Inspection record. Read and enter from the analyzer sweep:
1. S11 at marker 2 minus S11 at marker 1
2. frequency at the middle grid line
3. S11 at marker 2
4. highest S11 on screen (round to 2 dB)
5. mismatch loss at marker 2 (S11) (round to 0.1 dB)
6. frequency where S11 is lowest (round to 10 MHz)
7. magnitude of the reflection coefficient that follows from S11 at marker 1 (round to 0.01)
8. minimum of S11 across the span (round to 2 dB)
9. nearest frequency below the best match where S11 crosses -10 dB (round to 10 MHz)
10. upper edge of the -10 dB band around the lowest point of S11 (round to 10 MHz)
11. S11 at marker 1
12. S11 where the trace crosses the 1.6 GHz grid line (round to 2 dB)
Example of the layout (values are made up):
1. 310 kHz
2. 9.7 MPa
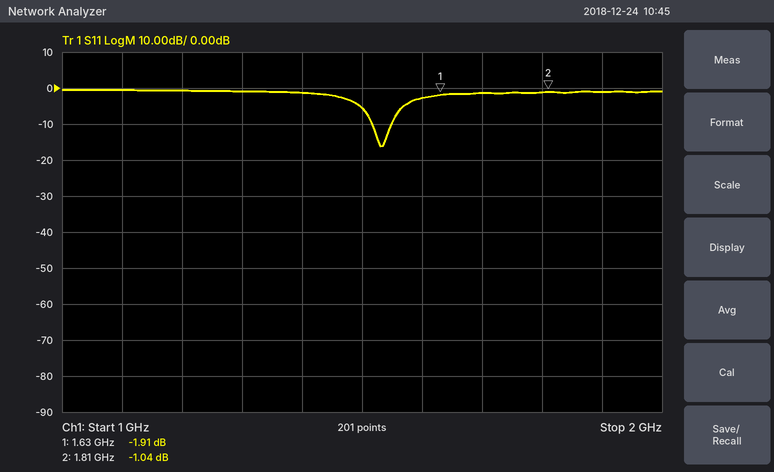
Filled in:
1. 0.87 dB
2. 1.5 GHz
3. -1.04 dB
4. 0 dB
5. 6.7 dB
6. 1.53 GHz
7. 0.80
8. -16 dB
9. 1.52 GHz
10. 1.55 GHz
11. -1.91 dB
12. -2 dB
